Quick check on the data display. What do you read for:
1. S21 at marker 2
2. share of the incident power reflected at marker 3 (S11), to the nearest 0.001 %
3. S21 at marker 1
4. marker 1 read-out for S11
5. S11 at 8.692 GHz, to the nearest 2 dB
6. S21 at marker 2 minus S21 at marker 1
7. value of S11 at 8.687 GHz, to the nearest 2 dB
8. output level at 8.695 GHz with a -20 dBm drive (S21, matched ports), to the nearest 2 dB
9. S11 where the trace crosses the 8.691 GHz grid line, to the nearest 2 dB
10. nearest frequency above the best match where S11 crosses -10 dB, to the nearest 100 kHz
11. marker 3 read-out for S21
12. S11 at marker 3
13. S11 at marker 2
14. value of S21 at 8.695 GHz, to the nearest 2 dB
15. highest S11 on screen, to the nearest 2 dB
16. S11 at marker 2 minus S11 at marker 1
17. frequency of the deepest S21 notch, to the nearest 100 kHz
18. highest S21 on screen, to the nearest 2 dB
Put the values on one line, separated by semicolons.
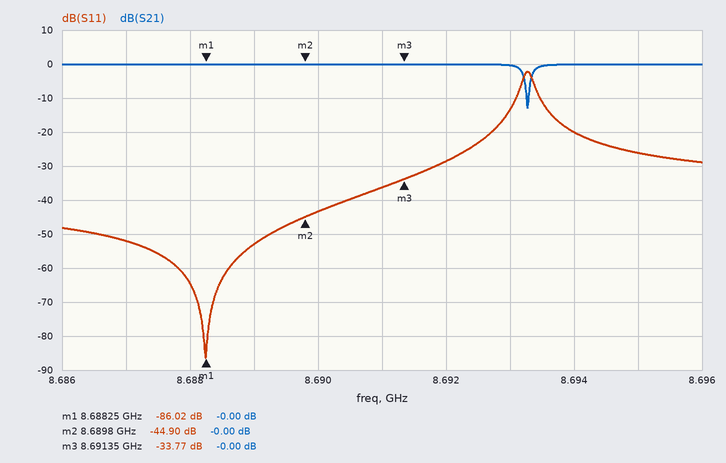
-0.00 dB; 0.042 %; -0.00 dB; -86.02 dB; -28 dB; 0.00 dB; -52 dB; -20 dBm; -36 dB; 8.6931 GHz; -0.00 dB; -33.77 dB; -44.90 dB; 0 dB; -2 dB; 41.12 dB; 8.6933 GHz; 0 dB
